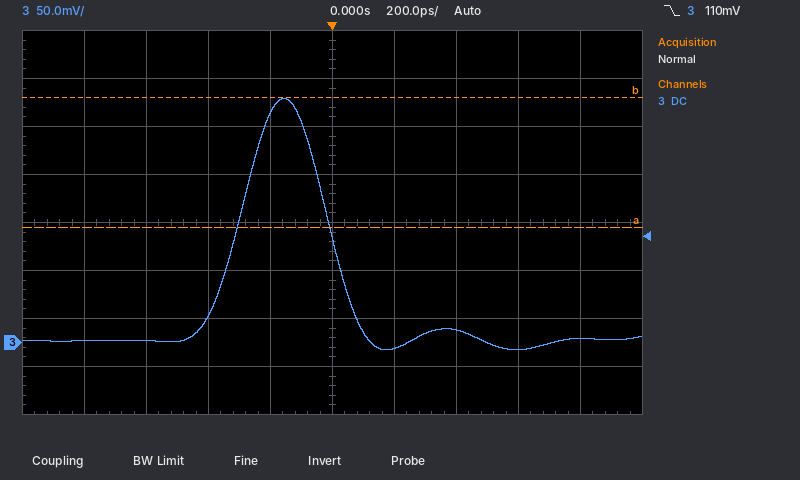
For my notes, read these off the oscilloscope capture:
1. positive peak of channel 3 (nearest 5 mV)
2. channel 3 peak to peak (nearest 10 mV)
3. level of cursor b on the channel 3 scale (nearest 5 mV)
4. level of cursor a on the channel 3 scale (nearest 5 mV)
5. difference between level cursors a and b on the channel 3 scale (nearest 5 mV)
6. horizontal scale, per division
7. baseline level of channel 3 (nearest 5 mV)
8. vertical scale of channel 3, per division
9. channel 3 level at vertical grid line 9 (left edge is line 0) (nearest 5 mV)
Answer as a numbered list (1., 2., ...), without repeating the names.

1. 255 mV
2. 260 mV
3. 255 mV
4. 120 mV
5. 135 mV
6. 200 ps
7. 0 mV
8. 50 mV
9. 5 mV
